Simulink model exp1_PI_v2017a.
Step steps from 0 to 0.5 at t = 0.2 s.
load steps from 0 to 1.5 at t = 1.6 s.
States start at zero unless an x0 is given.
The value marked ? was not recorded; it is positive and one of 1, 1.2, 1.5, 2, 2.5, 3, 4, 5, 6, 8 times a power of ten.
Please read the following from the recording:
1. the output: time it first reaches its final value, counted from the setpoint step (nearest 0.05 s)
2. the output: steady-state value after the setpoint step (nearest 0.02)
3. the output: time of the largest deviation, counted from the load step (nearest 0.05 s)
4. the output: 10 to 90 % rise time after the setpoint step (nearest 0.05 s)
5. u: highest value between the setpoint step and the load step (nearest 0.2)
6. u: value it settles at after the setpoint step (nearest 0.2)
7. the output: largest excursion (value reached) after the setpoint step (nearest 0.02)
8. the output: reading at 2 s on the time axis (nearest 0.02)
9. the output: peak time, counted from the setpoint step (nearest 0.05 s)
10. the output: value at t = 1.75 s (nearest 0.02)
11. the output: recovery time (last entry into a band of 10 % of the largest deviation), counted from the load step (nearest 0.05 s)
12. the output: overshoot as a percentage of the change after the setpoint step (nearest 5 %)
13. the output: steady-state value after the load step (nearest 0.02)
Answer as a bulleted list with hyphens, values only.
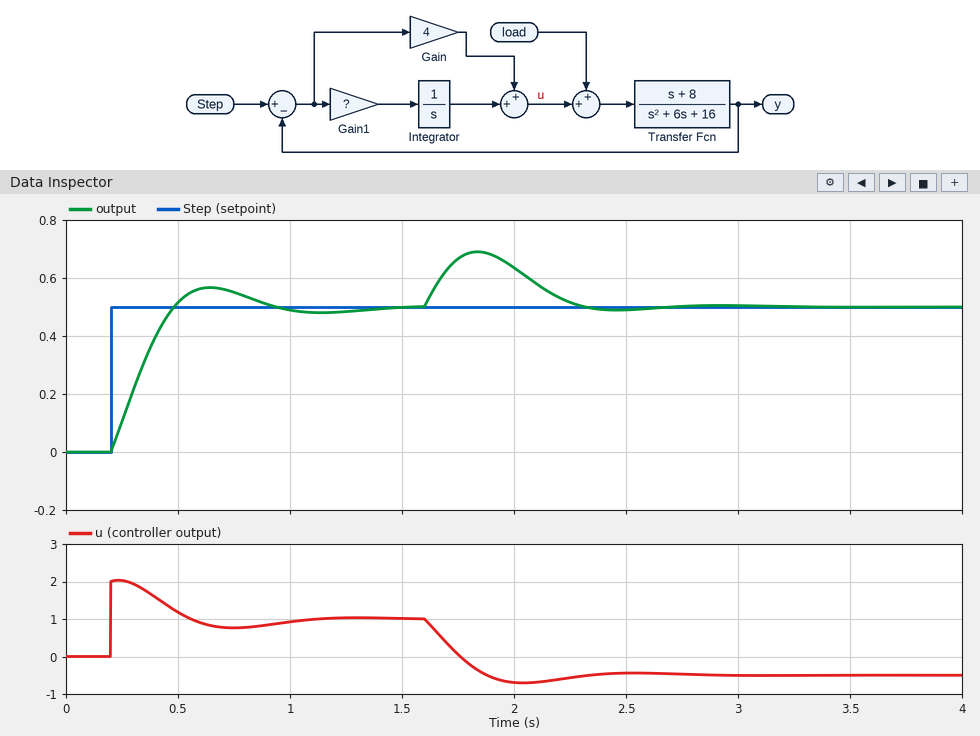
- 0.30 s
- 0.50
- 0.25 s
- 0.20 s
- 2.0
- 1.0
- 0.56
- 0.64
- 0.45 s
- 0.66
- 0.65 s
- 15 %
- 0.50
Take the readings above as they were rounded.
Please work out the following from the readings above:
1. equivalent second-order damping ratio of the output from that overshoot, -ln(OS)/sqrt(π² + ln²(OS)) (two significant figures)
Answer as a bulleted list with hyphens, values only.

- 0.52
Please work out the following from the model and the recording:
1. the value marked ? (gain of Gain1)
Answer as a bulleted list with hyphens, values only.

- 20
